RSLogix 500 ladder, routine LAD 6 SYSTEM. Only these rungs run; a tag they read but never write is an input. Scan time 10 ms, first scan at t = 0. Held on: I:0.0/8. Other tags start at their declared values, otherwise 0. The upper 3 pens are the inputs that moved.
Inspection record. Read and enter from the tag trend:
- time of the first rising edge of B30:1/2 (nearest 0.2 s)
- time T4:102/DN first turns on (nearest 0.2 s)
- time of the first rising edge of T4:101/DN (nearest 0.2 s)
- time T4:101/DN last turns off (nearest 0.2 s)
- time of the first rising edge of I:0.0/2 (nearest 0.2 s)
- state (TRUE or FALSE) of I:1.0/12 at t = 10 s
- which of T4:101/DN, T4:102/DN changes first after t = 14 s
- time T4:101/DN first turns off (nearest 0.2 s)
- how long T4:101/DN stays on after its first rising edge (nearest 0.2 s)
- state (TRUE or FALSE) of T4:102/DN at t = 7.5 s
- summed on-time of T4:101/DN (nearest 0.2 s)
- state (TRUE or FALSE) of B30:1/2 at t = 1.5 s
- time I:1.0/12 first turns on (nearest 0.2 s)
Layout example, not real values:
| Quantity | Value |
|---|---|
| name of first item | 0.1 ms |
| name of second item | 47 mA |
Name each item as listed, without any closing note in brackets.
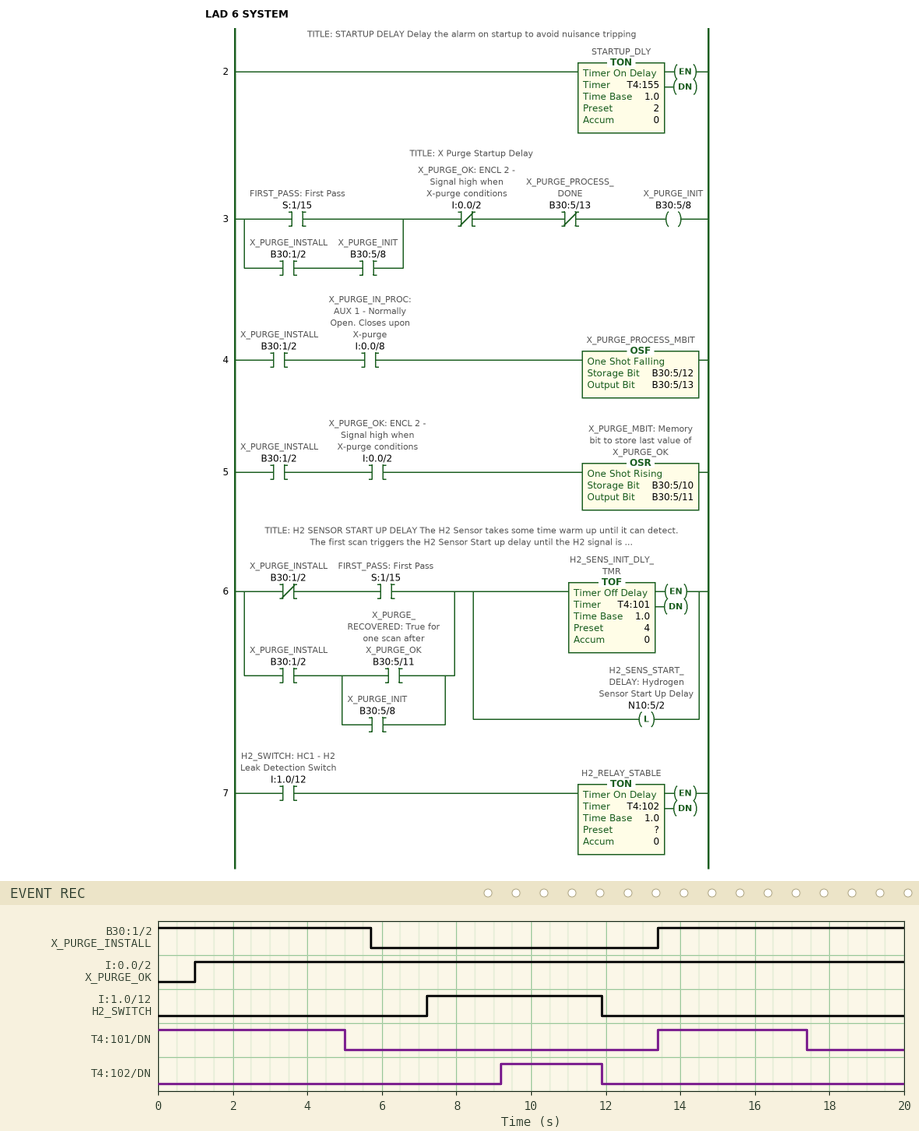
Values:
| Quantity | Value |
|---|---|
| time of the first rising edge of B30:1/2 | 13.4 s |
| time T4:102/DN first turns on | 9.2 s |
| time of the first rising edge of T4:101/DN | 13.4 s |
| time T4:101/DN last turns off | 17.4 s |
| time of the first rising edge of I:0.0/2 | 1.0 s |
| state (TRUE or FALSE) of I:1.0/12 at t = 10 s | TRUE |
| which of T4:101/DN, T4:102/DN changes first after t = 14 s | T4:101/DN |
| time T4:101/DN first turns off | 5.0 s |
| how long T4:101/DN stays on after its first rising edge | 4.0 s |
| state (TRUE or FALSE) of T4:102/DN at t = 7.5 s | FALSE |
| summed on-time of T4:101/DN | 9.0 s |
| state (TRUE or FALSE) of B30:1/2 at t = 1.5 s | TRUE |
| time I:1.0/12 first turns on | 7.2 s |
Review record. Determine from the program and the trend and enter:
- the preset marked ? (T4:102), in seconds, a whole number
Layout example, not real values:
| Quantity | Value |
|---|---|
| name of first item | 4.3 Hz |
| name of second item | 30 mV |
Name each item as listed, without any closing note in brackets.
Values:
| Quantity | Value |
|---|---|
| the preset marked ? (T4:102), in seconds, a whole number | 2 s |
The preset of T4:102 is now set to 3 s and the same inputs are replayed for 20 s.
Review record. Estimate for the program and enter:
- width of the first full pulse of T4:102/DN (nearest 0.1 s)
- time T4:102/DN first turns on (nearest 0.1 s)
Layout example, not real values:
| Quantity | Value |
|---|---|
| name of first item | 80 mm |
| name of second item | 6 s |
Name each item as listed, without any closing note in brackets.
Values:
| Quantity | Value |
|---|---|
| width of the first full pulse of T4:102/DN | 1.7 s |
| time T4:102/DN first turns on | 10.2 s |
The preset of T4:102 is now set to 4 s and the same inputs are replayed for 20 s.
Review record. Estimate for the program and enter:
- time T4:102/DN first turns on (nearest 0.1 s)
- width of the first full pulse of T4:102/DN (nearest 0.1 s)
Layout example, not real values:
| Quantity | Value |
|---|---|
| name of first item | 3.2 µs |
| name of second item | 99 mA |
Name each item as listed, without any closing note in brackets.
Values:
| Quantity | Value |
|---|---|
| time T4:102/DN first turns on | 11.2 s |
| width of the first full pulse of T4:102/DN | 0.7 s |
